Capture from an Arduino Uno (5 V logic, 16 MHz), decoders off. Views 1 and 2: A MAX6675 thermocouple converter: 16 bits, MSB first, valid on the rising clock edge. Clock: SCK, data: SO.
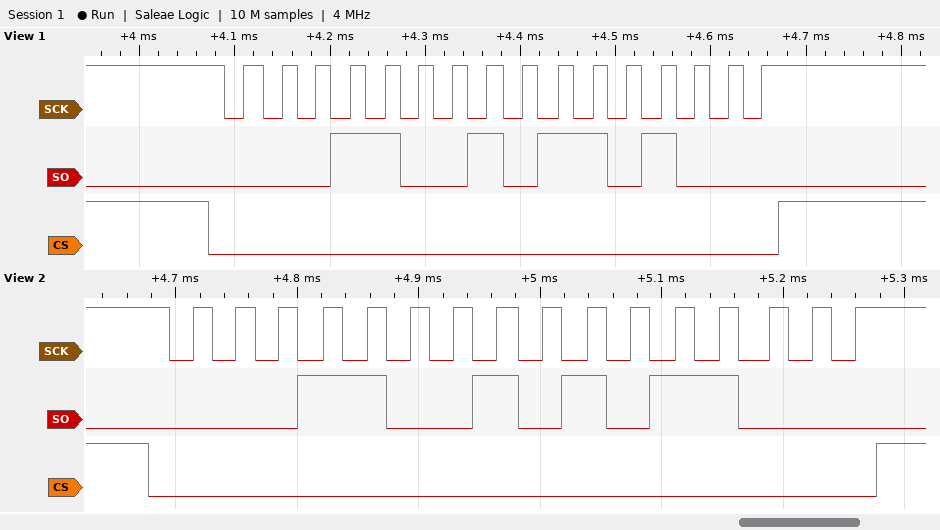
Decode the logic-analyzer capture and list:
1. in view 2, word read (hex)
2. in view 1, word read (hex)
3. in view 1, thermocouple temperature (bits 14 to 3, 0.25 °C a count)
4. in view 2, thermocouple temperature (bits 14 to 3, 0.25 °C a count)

0x1958
0x1968
203.25 °C
202.75 °C
